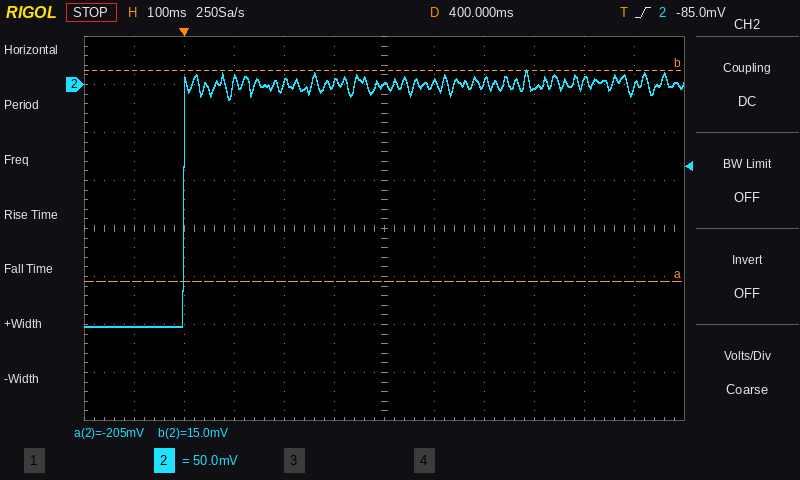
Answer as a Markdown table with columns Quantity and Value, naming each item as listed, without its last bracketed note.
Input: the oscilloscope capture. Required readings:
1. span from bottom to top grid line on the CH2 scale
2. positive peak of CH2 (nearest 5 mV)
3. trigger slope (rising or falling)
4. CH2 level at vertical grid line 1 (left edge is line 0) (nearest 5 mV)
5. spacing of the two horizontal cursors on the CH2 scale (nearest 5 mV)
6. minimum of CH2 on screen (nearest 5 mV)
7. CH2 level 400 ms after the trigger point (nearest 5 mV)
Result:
| Quantity | Value |
|---|---|
| span from bottom to top grid line on the CH2 scale | 400 mV |
| positive peak of CH2 | 15 mV |
| trigger slope | rising |
| CH2 level at vertical grid line 1 (left edge is line 0) | -250 mV |
| spacing of the two horizontal cursors on the CH2 scale | 220 mV |
| minimum of CH2 on screen | -250 mV |
| CH2 level 400 ms after the trigger point | 0 mV |
